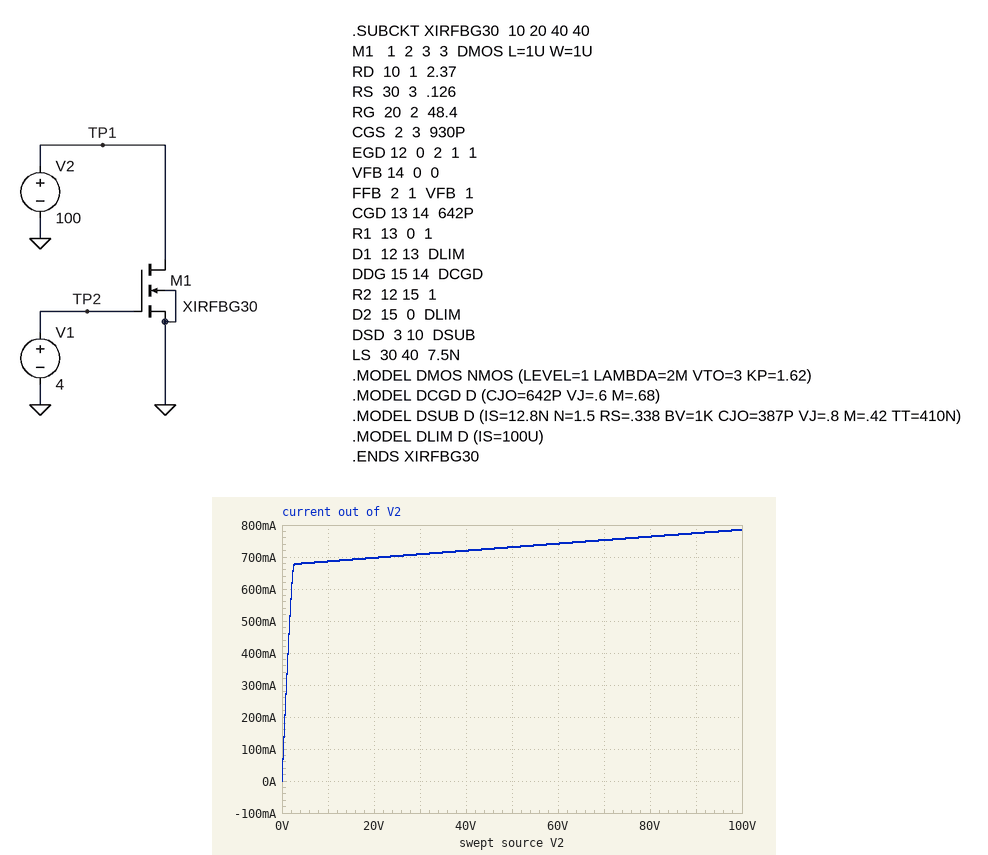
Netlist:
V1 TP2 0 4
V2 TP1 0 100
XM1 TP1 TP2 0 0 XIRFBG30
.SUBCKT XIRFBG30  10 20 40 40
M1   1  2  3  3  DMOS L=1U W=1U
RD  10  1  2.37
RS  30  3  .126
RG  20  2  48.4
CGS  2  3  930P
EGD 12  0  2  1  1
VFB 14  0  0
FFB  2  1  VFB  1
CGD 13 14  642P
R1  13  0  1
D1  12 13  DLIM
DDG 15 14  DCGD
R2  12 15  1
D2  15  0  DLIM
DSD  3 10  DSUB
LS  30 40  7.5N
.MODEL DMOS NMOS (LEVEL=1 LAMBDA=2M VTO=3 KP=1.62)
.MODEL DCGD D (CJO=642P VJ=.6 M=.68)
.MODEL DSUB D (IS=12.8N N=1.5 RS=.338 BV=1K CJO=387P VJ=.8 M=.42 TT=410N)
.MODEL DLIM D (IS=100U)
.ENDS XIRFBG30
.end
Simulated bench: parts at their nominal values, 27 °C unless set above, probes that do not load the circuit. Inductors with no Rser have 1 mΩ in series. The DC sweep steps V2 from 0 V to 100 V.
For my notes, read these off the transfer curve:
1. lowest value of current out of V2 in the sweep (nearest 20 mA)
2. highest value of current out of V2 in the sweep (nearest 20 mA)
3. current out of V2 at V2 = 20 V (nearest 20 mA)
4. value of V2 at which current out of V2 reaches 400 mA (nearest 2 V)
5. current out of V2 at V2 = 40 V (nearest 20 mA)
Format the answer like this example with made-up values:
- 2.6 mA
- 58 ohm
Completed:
- 0 A
- 780 mA
- 700 mA
- 2 V
- 720 mA
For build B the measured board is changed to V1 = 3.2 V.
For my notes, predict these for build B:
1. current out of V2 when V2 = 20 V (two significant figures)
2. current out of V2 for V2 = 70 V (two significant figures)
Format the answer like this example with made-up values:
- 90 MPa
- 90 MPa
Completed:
- 32 mA
- 35 mA
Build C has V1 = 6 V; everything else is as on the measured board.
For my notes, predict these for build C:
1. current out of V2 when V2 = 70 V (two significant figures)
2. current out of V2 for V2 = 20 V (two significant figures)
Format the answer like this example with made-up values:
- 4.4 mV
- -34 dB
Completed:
- 5.0 A
- 4.7 A
